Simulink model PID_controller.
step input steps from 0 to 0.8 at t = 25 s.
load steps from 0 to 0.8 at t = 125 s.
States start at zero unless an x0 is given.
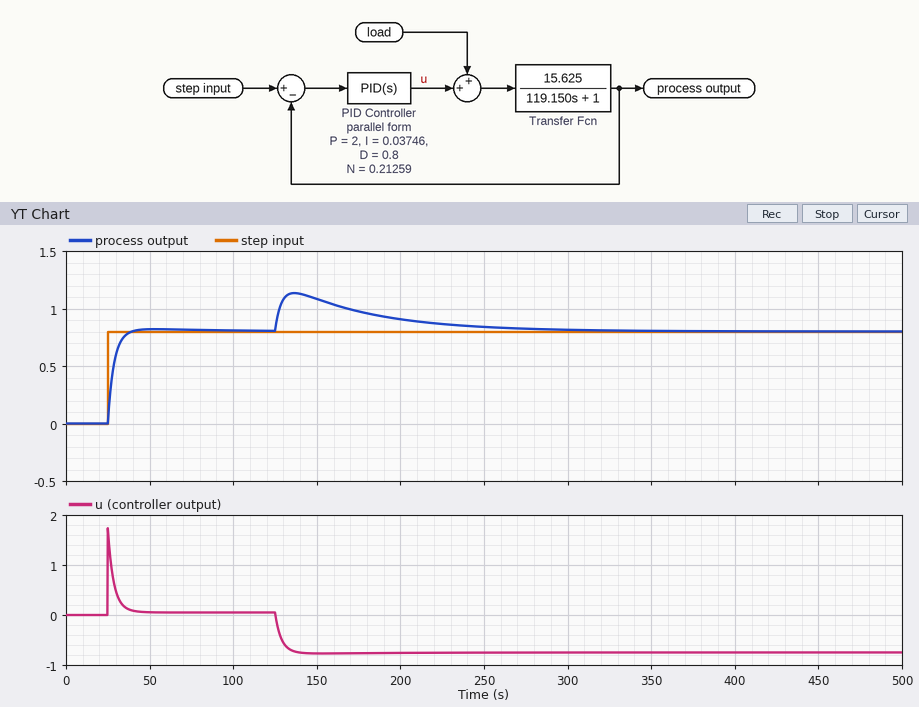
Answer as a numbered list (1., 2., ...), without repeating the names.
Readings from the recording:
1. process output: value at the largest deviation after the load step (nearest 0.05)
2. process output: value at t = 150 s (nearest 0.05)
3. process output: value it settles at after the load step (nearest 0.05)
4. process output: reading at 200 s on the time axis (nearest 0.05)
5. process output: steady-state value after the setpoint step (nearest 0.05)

1. 1.15
2. 1.10
3. 0.80
4. 0.90
5. 0.80
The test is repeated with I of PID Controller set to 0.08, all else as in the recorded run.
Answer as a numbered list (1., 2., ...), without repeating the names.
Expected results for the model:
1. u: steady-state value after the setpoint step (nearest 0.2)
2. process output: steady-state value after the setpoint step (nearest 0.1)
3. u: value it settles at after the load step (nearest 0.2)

1. 0.0
2. 0.8
3. -0.8
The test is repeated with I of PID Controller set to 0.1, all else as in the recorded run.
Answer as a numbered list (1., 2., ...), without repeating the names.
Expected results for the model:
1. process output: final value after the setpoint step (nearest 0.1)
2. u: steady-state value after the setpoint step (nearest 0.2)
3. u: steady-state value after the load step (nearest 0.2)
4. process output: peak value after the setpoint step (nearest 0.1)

1. 0.8
2. 0.0
3. -0.8
4. 0.9
